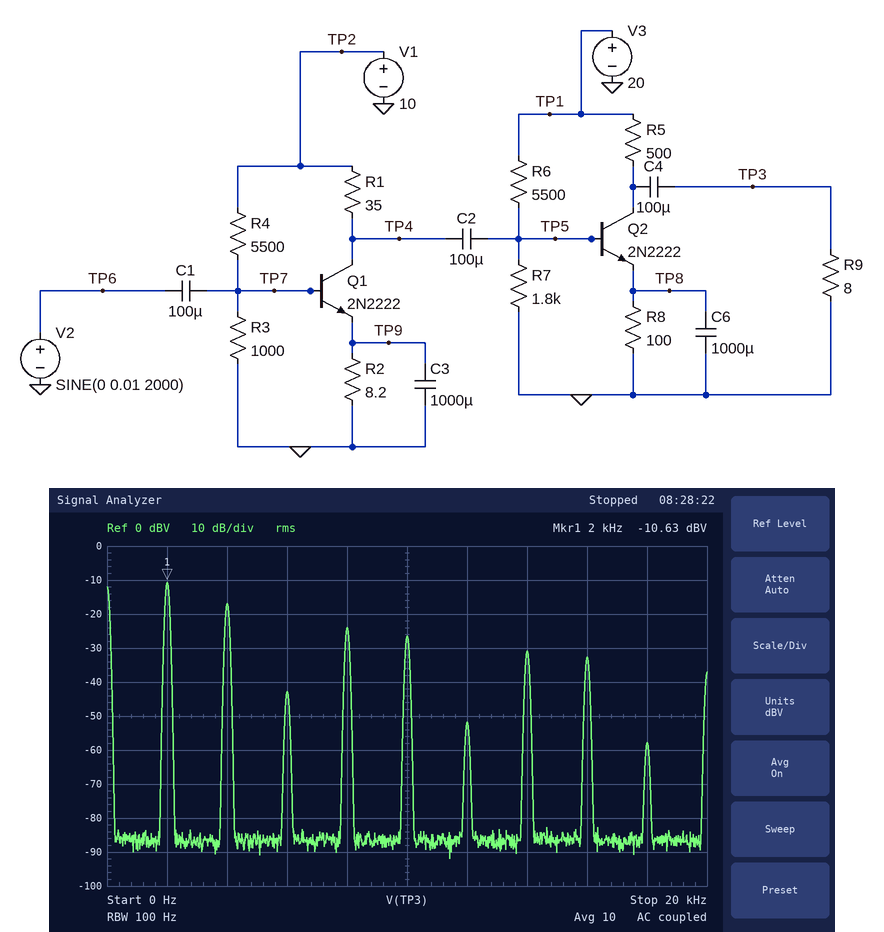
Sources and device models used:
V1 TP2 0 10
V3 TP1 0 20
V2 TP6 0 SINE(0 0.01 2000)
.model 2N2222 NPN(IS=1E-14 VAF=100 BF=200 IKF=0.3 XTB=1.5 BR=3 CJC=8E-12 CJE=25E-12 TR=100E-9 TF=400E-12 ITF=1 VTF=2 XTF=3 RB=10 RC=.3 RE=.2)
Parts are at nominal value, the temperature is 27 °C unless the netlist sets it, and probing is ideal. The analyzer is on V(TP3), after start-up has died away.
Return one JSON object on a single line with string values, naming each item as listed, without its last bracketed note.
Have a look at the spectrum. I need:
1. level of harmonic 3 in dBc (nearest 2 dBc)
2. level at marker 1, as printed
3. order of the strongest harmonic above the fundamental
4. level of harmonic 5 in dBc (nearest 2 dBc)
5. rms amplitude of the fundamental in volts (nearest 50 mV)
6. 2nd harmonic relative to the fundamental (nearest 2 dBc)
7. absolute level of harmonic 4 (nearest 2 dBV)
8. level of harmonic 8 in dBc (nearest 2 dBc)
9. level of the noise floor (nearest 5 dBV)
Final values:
{"level of harmonic 3 in dBc": "-32 dBc", "level at marker 1, as printed": "-10.63 dBV", "order of the strongest harmonic above the fundamental": "2", "level of harmonic 5 in dBc": "-16 dBc", "rms amplitude of the fundamental in volts": "300 mV", "2nd harmonic relative to the fundamental": "-6 dBc", "absolute level of harmonic 4": "-24 dBV", "level of harmonic 8 in dBc": "-22 dBc", "level of the noise floor": "-85 dBV"}
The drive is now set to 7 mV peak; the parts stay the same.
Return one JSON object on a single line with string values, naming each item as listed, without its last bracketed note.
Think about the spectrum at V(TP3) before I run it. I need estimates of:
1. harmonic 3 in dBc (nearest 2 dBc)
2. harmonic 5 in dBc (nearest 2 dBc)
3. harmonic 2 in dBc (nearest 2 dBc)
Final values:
{"harmonic 3 in dBc": "-20 dBc", "harmonic 5 in dBc": "-22 dBc", "harmonic 2 in dBc": "-8 dBc"}
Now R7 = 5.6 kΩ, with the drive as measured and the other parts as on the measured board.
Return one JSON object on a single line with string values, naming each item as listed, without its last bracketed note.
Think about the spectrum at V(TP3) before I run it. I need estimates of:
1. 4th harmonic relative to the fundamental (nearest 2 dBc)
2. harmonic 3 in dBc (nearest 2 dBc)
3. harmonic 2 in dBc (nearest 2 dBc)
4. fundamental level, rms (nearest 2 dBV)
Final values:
{"4th harmonic relative to the fundamental": "-20 dBc", "harmonic 3 in dBc": "-10 dBc", "harmonic 2 in dBc": "-18 dBc", "fundamental level, rms": "-12 dBV"}
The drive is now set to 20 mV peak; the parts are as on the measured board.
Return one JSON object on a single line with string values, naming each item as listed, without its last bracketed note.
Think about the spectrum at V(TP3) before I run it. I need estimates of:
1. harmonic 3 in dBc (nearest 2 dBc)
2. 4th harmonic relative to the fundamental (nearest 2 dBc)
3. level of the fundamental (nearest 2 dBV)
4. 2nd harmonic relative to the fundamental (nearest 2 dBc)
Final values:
{"harmonic 3 in dBc": "-16 dBc", "4th harmonic relative to the fundamental": "-16 dBc", "level of the fundamental": "-10 dBV", "2nd harmonic relative to the fundamental": "-4 dBc"}
